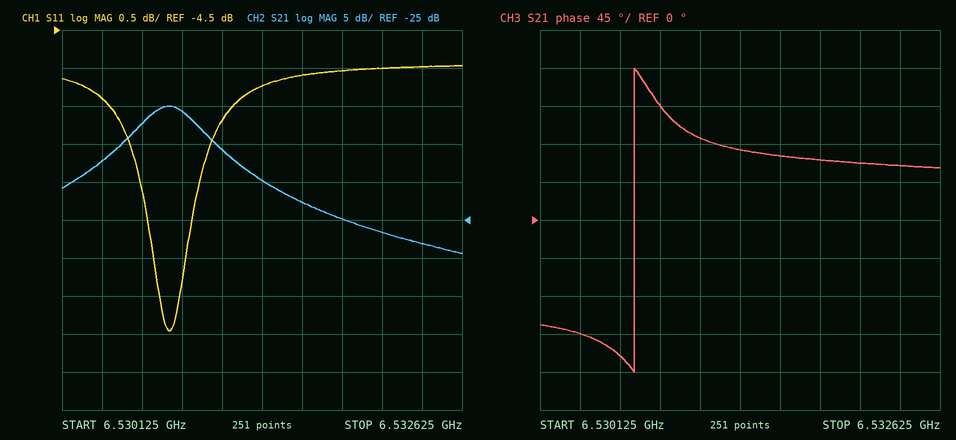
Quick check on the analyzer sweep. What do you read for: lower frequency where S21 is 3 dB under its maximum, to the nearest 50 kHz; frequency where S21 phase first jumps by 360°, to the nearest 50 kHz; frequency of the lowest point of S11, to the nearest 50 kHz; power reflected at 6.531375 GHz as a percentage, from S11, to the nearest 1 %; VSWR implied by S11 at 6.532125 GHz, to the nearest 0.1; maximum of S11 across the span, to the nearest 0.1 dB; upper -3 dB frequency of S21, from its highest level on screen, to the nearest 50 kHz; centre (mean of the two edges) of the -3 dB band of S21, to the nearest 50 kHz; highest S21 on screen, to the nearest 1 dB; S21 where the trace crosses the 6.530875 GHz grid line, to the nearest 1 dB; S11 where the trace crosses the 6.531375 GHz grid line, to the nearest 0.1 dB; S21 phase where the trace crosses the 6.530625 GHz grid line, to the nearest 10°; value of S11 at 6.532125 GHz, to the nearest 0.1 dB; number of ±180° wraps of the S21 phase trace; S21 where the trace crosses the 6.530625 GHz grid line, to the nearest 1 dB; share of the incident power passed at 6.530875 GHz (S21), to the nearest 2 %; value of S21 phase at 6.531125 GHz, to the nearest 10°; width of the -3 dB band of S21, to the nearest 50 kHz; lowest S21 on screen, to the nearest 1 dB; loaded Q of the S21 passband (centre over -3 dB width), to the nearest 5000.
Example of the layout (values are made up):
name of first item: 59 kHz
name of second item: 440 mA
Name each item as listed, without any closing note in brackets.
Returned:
lower frequency where S21 is 3 dB under its maximum, to the nearest 50 kHz: 6.53060 GHz
frequency where S21 phase first jumps by 360°, to the nearest 50 kHz: 6.53070 GHz
frequency of the lowest point of S11, to the nearest 50 kHz: 6.53080 GHz
power reflected at 6.531375 GHz as a percentage, from S11, to the nearest 1 %: 30 %
VSWR implied by S11 at 6.532125 GHz, to the nearest 0.1: 3.6
maximum of S11 across the span, to the nearest 0.1 dB: -5.0 dB
upper -3 dB frequency of S21, from its highest level on screen, to the nearest 50 kHz: 6.53100 GHz
centre (mean of the two edges) of the -3 dB band of S21, to the nearest 50 kHz: 6.53080 GHz
highest S21 on screen, to the nearest 1 dB: -10 dB
S21 where the trace crosses the 6.530875 GHz grid line, to the nearest 1 dB: -11 dB
S11 where the trace crosses the 6.531375 GHz grid line, to the nearest 0.1 dB: -5.2 dB
S21 phase where the trace crosses the 6.530625 GHz grid line, to the nearest 10°: -160°
value of S11 at 6.532125 GHz, to the nearest 0.1 dB: -5.0 dB
number of ±180° wraps of the S21 phase trace: 1
S21 where the trace crosses the 6.530625 GHz grid line, to the nearest 1 dB: -12 dB
share of the incident power passed at 6.530875 GHz (S21), to the nearest 2 %: 8 %
value of S21 phase at 6.531125 GHz, to the nearest 10°: 100°
width of the -3 dB band of S21, to the nearest 50 kHz: 400 kHz
lowest S21 on screen, to the nearest 1 dB: -29 dB
loaded Q of the S21 passband (centre over -3 dB width), to the nearest 5000: 15000
